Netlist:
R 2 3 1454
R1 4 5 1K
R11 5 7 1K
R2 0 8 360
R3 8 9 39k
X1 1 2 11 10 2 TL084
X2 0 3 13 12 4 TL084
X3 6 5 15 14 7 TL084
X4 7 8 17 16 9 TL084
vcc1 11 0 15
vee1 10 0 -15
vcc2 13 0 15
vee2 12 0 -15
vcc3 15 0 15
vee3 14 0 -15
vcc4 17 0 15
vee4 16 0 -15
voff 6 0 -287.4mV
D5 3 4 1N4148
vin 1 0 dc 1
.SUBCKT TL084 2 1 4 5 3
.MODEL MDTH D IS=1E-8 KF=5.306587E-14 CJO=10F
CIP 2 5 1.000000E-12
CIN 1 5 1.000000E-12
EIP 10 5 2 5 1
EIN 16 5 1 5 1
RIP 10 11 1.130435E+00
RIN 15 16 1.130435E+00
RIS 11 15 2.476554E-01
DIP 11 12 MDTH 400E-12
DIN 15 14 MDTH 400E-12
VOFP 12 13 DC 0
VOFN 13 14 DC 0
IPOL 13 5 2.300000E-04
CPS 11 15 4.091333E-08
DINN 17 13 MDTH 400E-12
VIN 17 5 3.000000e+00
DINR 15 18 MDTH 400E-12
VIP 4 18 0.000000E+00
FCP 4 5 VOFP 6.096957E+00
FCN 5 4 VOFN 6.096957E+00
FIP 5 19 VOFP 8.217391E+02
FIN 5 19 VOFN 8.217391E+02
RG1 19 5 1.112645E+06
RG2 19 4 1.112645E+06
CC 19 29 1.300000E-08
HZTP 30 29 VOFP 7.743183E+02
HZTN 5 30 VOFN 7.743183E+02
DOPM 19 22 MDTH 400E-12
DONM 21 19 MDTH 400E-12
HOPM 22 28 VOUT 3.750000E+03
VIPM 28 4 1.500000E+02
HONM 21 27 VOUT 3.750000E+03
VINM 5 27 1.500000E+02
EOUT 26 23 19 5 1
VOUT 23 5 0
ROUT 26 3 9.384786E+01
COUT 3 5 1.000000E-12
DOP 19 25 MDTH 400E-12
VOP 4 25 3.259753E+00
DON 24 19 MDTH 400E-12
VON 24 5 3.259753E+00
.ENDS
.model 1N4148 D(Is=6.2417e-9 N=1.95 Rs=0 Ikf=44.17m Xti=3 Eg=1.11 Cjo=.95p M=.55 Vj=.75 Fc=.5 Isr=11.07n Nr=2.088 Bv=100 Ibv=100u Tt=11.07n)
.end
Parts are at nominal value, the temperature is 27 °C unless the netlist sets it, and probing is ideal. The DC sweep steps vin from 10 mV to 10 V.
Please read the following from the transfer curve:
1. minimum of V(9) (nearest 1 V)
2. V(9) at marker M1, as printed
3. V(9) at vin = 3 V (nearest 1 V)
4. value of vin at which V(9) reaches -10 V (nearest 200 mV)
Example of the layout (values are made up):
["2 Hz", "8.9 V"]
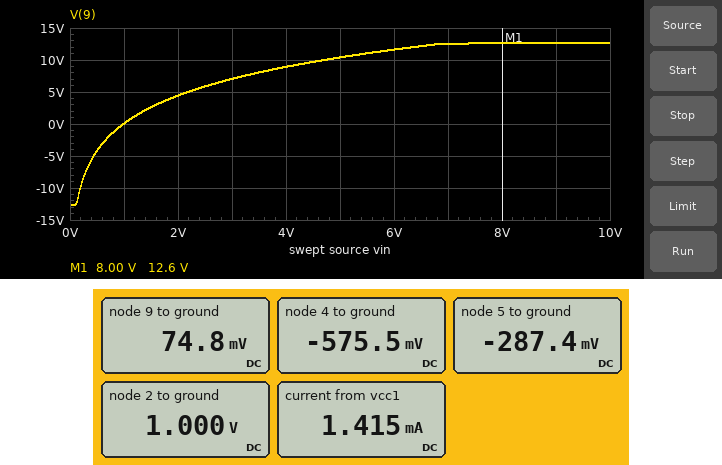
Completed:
["-13 V", "12.6 V", "7 V", "200 mV"]
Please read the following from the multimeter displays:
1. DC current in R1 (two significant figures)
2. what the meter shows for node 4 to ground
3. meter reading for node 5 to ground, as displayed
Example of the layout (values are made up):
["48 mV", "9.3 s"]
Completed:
["290 µA", "-575.5 mV", "-287.4 mV"]
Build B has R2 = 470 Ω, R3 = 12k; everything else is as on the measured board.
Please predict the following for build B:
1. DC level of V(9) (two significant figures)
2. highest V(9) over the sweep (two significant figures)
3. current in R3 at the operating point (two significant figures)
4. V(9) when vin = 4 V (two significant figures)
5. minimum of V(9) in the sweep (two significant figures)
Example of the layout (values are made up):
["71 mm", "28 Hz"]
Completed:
["18 mV", "3.7 V", "1.5 µA", "2.2 V", "-6.7 V"]
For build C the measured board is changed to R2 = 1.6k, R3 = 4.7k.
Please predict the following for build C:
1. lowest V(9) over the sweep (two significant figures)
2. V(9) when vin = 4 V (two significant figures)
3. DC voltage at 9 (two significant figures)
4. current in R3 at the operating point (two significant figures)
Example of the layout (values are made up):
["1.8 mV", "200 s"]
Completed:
["-990 mV", "320 mV", "2.7 mV", "430 nA"]
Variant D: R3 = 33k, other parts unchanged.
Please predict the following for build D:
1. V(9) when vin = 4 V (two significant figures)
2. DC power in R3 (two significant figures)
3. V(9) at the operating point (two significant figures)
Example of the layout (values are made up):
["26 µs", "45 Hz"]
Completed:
["7.6 V", "120 nW", "63 mV"]
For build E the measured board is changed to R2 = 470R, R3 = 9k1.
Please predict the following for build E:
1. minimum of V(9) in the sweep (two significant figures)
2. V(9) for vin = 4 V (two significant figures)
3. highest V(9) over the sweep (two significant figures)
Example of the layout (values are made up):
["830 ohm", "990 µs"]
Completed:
["-5.1 V", "1.7 V", "2.8 V"]
